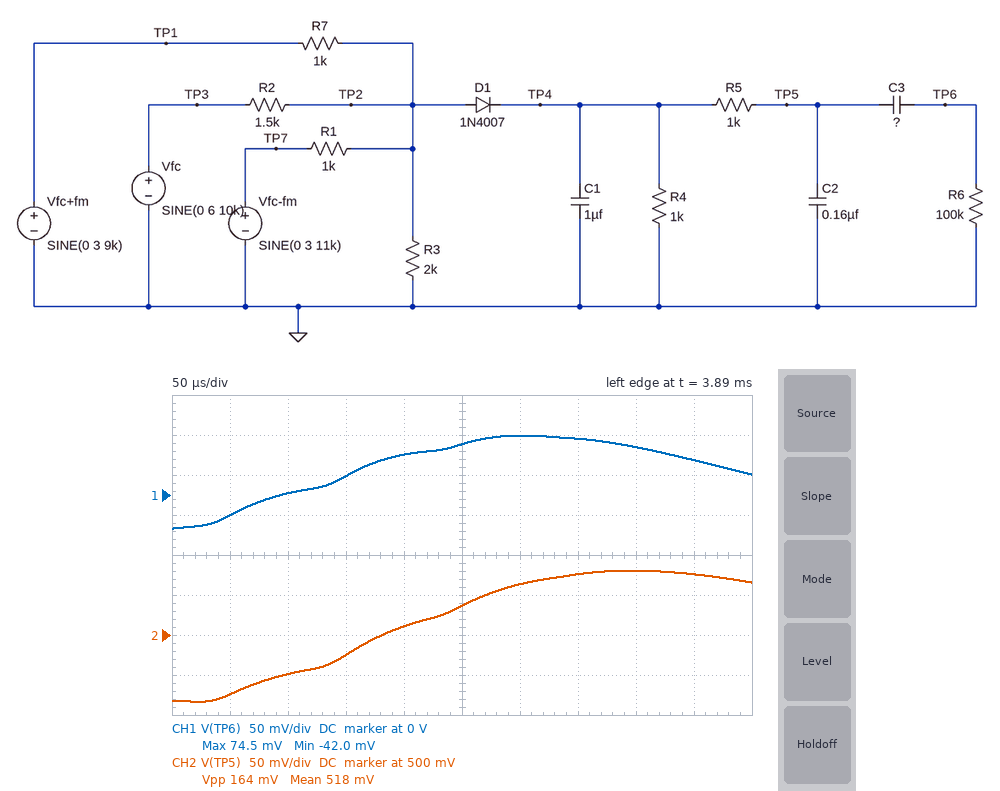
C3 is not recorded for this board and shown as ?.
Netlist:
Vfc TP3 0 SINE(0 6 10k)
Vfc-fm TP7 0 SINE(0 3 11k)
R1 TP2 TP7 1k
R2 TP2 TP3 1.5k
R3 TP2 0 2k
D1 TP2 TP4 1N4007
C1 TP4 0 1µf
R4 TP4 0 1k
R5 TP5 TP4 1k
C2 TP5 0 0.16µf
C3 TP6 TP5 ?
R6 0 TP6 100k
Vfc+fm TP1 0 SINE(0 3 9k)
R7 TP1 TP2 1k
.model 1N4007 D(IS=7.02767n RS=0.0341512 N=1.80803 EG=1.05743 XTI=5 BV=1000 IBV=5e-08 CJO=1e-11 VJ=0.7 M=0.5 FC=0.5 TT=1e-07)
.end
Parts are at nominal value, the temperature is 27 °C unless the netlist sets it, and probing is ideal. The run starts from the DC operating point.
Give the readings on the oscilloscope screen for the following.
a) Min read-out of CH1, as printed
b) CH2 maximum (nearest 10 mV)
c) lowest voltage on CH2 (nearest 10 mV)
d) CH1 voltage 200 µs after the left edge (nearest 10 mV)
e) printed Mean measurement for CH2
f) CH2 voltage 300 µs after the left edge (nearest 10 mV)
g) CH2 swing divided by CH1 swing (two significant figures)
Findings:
-42.0 mV
580 mV
420 mV
50 mV
518 mV
560 mV
1.4
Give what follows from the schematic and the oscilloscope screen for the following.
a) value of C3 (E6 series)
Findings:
2.2 nF
